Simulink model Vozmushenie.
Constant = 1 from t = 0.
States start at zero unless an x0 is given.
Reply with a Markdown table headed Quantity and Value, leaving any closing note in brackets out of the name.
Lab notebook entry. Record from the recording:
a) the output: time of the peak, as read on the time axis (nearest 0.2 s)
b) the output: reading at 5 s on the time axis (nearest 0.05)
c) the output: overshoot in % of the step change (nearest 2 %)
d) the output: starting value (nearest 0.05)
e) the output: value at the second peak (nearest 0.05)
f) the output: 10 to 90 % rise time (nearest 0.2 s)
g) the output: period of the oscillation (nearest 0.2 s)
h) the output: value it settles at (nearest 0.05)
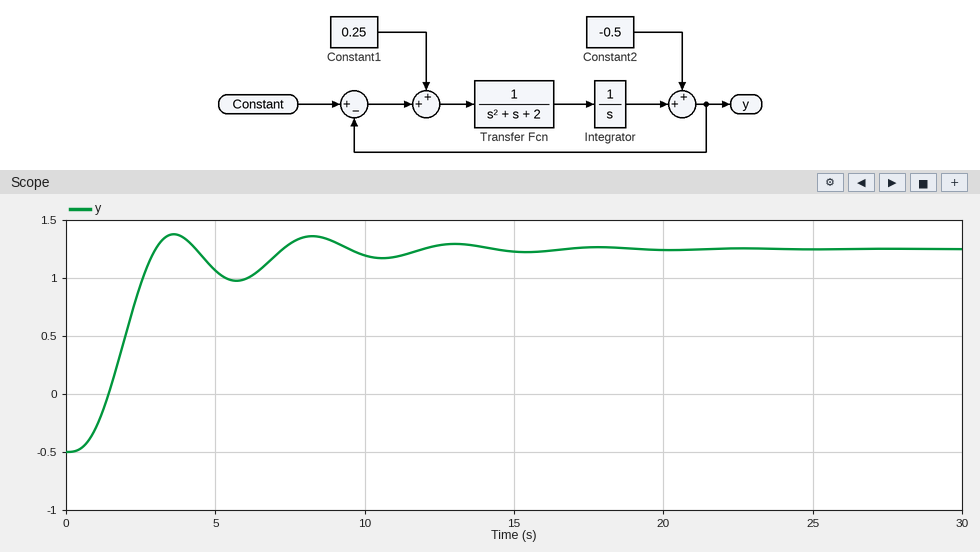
| Quantity | Value |
|---|---|
| the output: time of the peak, as read on the time axis | 3.6 s |
| the output: reading at 5 s on the time axis | 1.05 |
| the output: overshoot in % of the step change | 8 % |
| the output: starting value | -0.50 |
| the output: value at the second peak | 1.35 |
| the output: 10 to 90 % rise time | 1.8 s |
| the output: period of the oscillation | 4.6 s |
| the output: value it settles at | 1.25 |
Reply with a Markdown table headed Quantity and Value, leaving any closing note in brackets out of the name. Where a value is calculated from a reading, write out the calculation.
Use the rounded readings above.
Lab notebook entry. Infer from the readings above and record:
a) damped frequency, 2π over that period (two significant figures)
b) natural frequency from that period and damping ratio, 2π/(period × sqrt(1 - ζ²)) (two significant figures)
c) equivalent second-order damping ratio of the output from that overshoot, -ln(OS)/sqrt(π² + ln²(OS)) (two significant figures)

| Quantity | Value |
|---|---|
| damped frequency, 2π over that period | 2π / 4.6 = 1.4 rad/s |
| natural frequency from that period and damping ratio, 2π/(period × sqrt(1 - ζ²)) | 2π / (4.6 × sqrt(1 - 0.63²)) = 1.8 rad/s |
| equivalent second-order damping ratio of the output from that overshoot, -ln(OS)/sqrt(π² + ln²(OS)) | ln(0.08) = -2.526; 2.526 / sqrt(9.870 + 6.379) = 0.63 |
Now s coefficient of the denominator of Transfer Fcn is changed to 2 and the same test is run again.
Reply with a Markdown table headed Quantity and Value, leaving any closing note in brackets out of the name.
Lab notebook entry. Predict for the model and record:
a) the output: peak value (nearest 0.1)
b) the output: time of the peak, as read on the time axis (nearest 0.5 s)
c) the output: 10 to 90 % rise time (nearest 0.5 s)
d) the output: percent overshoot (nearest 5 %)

| Quantity | Value |
|---|---|
| the output: peak value | 1.4 |
| the output: time of the peak, as read on the time axis | 5.0 s |
| the output: 10 to 90 % rise time | 2.5 s |
| the output: percent overshoot | 10 % |
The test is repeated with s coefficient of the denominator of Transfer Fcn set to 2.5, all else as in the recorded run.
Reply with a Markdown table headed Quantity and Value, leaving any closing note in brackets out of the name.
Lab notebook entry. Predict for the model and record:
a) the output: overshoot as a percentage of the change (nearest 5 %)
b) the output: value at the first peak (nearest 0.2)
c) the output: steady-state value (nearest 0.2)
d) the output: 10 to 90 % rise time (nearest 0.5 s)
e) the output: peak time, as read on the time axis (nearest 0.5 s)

| Quantity | Value |
|---|---|
| the output: overshoot as a percentage of the change | 10 % |
| the output: value at the first peak | 1.4 |
| the output: steady-state value | 1.2 |
| the output: 10 to 90 % rise time | 2.5 s |
| the output: peak time, as read on the time axis | 5.5 s |
